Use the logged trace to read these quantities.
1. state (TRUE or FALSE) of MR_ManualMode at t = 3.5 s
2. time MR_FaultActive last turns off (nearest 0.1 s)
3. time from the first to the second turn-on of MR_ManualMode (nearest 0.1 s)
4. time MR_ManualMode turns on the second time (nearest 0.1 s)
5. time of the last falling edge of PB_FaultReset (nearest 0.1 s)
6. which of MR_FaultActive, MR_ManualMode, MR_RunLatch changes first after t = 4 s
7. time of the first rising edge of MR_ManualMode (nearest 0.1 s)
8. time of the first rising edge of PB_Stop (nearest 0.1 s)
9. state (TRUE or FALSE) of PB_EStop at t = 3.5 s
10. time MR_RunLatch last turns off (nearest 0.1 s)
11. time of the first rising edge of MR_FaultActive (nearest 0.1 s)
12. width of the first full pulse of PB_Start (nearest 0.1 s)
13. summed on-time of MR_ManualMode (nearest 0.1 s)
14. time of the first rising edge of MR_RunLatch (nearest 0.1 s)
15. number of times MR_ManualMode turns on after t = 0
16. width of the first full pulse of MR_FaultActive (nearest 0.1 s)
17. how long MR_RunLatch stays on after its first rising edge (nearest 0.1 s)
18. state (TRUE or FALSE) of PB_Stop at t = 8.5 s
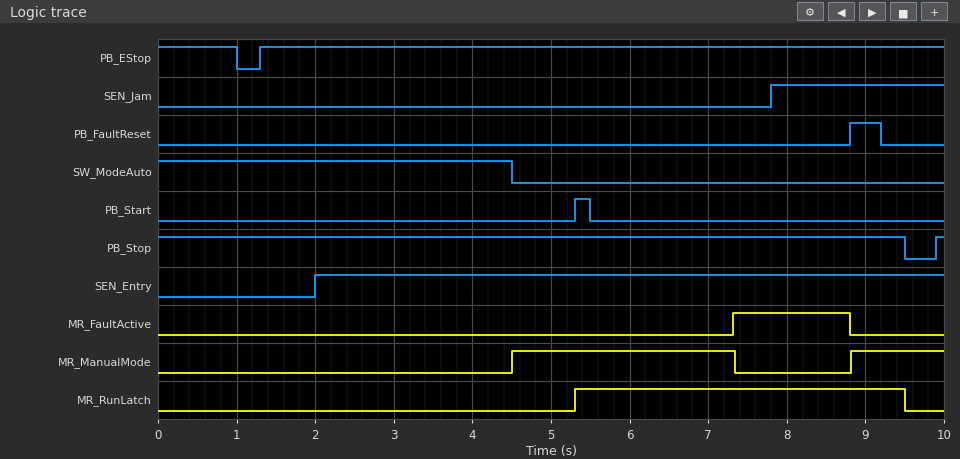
FALSE
8.8 s
4.3 s
8.8 s
9.2 s
MR_ManualMode
4.5 s
9.9 s
TRUE
9.5 s
7.3 s
0.2 s
4.0 s
5.3 s
2
1.5 s
4.2 s
TRUE
